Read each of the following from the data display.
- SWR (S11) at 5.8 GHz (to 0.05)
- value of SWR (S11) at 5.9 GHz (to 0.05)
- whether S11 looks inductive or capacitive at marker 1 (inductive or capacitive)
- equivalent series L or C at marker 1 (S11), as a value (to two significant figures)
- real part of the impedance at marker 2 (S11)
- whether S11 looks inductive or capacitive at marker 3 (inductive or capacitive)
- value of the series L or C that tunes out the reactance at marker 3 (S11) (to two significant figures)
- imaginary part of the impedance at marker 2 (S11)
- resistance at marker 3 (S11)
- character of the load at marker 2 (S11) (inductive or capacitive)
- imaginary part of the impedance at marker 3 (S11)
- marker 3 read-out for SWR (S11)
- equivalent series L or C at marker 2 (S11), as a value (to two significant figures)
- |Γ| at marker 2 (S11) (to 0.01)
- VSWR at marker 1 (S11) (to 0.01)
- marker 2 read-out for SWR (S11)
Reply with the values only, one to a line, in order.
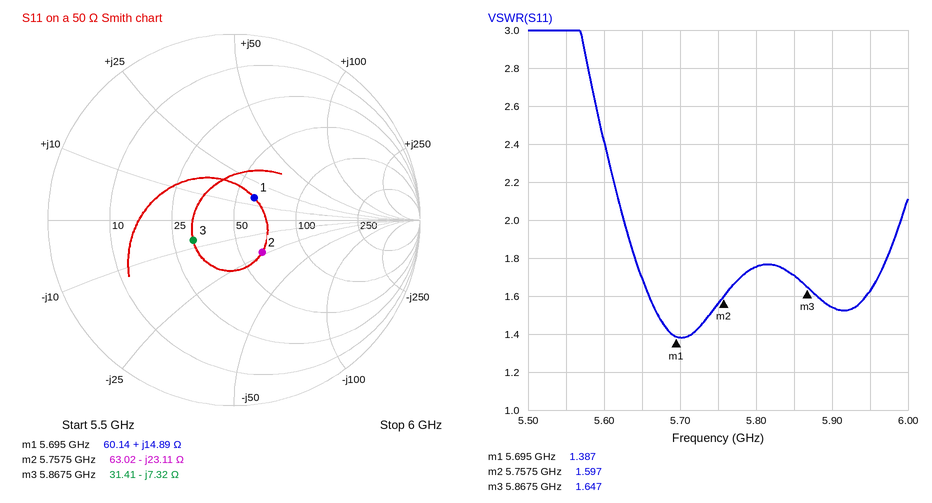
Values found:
1.75
1.55
inductive
420 pH
63.02 Ω
capacitive
200 pH
-23.11 Ω
31.41 Ω
capacitive
-7.32 Ω
1.647
1.2 pF
0.23
1.39
1.597
